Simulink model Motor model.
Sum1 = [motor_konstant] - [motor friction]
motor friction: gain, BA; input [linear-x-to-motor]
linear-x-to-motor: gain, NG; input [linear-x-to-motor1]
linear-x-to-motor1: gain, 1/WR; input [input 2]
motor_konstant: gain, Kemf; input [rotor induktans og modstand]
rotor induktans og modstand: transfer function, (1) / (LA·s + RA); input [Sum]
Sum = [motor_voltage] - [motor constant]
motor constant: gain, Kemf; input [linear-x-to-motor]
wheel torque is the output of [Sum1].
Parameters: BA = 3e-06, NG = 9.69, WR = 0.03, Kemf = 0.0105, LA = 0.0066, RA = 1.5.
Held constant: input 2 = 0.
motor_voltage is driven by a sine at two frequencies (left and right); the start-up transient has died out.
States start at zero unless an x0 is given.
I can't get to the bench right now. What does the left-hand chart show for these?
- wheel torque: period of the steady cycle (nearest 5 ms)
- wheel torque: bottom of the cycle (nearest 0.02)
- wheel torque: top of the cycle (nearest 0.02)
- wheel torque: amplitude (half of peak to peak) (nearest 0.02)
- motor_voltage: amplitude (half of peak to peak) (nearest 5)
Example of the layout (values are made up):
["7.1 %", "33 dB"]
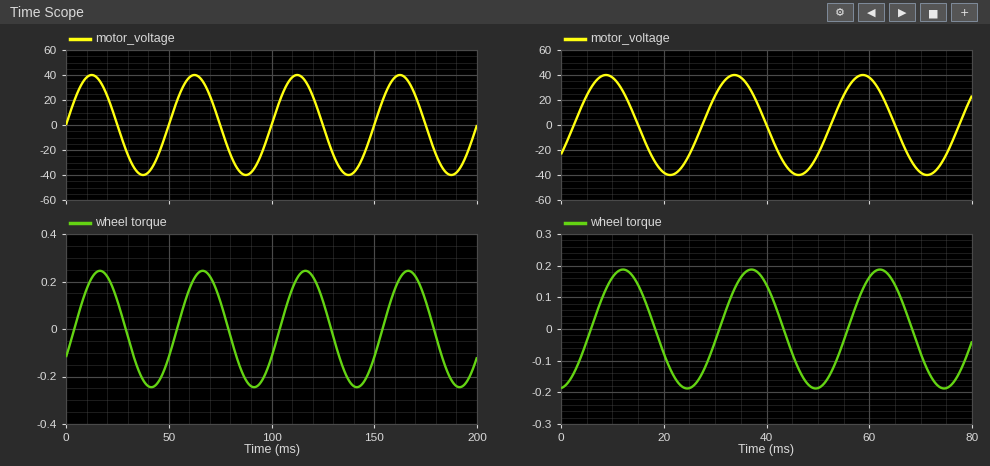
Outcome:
["50 ms", "-0.24", "0.24", "0.24", "40"]
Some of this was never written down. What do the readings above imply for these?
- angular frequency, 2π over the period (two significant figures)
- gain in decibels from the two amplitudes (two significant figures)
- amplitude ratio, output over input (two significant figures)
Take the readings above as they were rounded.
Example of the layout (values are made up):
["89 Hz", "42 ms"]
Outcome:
["0.13 rad/ms", "-44 dB", "0.0060"]
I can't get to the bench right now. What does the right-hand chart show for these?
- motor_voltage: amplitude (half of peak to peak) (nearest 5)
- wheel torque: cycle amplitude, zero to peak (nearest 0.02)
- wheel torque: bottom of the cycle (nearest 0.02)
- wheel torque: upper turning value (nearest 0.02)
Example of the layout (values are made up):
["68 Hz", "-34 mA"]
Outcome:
["40", "0.18", "-0.18", "0.18"]
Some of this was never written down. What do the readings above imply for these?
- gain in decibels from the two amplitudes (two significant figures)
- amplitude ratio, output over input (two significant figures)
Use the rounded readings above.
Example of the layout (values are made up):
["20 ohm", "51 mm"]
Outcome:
["-47 dB", "0.0045"]
